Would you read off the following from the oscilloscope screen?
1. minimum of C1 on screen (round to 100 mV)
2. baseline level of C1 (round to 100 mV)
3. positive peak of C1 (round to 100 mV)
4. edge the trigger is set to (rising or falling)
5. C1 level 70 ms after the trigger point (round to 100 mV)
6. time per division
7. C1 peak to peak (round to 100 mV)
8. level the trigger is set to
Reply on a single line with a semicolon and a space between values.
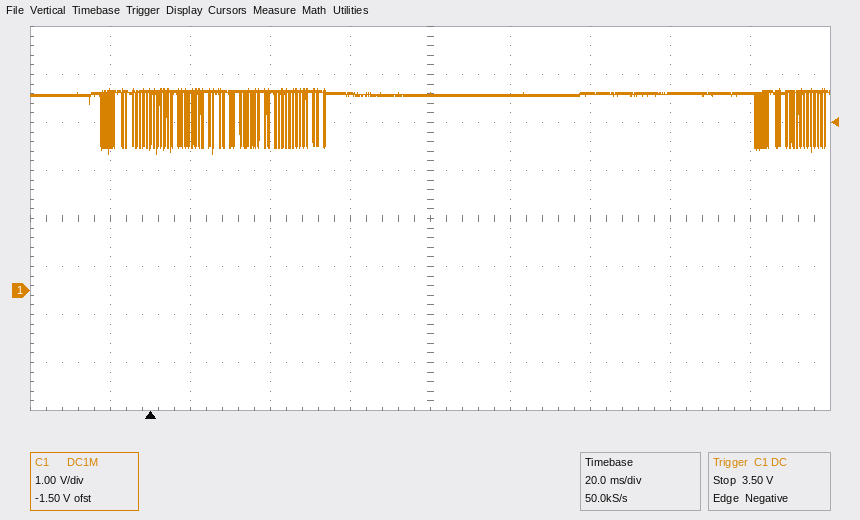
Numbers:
2.8 V; 4.1 V; 4.2 V; falling; 4.1 V; 20 ms; 1.4 V; 3.50 V
